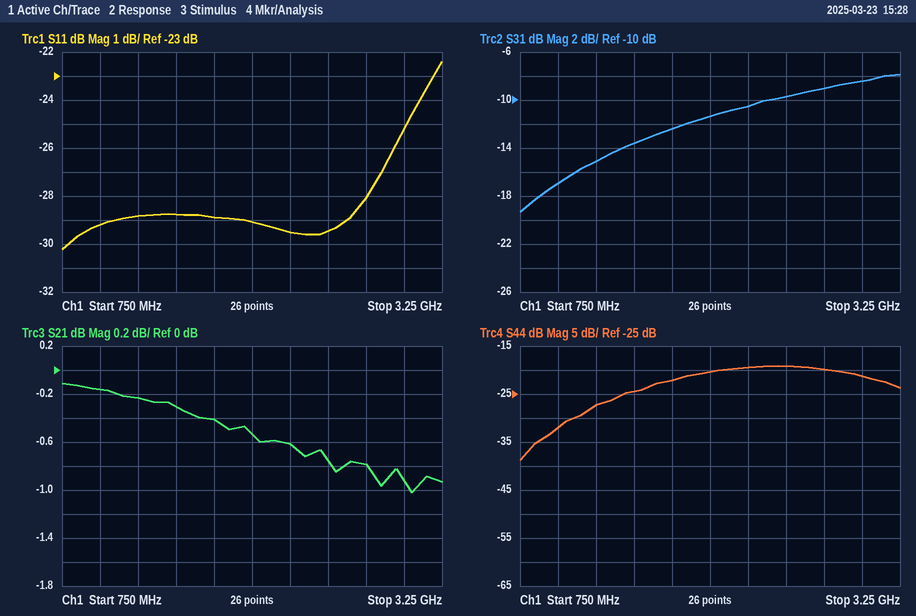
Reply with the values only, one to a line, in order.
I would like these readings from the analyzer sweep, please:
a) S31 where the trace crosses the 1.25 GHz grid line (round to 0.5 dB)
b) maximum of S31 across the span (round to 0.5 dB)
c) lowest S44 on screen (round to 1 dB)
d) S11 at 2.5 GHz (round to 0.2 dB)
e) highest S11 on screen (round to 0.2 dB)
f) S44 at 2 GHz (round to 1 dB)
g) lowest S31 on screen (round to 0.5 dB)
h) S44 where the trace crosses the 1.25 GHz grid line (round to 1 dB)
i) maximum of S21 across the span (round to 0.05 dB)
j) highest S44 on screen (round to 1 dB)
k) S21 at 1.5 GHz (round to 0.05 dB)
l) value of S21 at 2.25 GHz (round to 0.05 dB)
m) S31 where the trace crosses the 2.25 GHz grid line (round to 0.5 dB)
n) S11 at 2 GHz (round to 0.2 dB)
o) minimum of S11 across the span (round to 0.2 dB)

-15.0 dB
-8.0 dB
-39 dB
-29.4 dB
-22.4 dB
-20 dB
-19.5 dB
-27 dB
-0.10 dB
-19 dB
-0.30 dB
-0.60 dB
-10.5 dB
-29.0 dB
-30.2 dB
